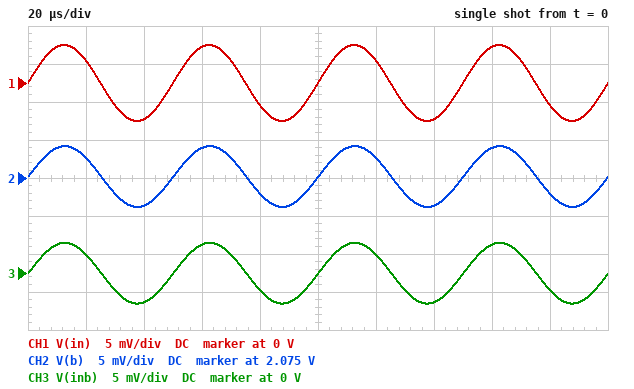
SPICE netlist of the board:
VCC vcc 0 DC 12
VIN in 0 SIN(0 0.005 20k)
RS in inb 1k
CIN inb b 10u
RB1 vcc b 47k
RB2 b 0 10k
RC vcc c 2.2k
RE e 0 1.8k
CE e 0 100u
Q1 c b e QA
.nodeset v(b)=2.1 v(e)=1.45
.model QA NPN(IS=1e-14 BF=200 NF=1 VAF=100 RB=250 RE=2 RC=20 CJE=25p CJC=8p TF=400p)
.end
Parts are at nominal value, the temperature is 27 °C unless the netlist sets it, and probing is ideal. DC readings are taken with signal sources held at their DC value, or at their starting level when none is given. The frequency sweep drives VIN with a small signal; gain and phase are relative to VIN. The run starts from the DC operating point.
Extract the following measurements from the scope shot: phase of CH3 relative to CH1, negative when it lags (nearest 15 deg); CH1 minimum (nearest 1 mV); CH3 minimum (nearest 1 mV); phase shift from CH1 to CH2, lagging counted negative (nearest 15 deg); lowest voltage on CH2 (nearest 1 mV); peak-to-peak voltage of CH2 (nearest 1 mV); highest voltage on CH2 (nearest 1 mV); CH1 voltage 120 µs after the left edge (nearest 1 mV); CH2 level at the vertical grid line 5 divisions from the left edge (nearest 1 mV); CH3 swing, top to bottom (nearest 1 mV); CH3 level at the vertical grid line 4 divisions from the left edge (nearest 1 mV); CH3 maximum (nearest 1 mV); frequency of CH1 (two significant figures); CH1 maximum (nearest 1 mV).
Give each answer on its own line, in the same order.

0 deg
-5 mV
-4 mV
0 deg
2.071 V
8 mV
2.079 V
3 mV
2.075 V
8 mV
-2 mV
4 mV
20 kHz
5 mV
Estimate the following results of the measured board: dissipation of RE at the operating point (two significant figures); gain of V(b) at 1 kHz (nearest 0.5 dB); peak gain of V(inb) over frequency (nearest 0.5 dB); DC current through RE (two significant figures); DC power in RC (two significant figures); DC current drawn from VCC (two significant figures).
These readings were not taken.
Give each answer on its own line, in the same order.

1.1 mW
-2.0 dB
0 dB
790 µA
1.4 mW
1.0 mA
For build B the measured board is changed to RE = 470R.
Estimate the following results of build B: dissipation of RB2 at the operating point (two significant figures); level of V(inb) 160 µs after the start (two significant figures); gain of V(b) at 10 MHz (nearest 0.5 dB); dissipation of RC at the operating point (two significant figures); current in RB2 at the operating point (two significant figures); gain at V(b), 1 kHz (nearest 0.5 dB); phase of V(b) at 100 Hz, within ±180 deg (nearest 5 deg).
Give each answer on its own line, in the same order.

400 µW
3.0 mV
-14.0 dB
17 mW
200 µA
-3.5 dB
-5 deg
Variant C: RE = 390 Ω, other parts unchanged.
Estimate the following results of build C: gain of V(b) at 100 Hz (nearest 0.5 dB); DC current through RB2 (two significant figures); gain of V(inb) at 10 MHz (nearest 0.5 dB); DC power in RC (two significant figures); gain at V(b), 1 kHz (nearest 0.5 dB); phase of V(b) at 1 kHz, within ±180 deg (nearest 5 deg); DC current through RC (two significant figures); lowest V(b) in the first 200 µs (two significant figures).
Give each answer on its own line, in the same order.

-2.5 dB
200 µA
-14.0 dB
23 mW
-4.0 dB
0 deg
3.3 mA
2.0 V
